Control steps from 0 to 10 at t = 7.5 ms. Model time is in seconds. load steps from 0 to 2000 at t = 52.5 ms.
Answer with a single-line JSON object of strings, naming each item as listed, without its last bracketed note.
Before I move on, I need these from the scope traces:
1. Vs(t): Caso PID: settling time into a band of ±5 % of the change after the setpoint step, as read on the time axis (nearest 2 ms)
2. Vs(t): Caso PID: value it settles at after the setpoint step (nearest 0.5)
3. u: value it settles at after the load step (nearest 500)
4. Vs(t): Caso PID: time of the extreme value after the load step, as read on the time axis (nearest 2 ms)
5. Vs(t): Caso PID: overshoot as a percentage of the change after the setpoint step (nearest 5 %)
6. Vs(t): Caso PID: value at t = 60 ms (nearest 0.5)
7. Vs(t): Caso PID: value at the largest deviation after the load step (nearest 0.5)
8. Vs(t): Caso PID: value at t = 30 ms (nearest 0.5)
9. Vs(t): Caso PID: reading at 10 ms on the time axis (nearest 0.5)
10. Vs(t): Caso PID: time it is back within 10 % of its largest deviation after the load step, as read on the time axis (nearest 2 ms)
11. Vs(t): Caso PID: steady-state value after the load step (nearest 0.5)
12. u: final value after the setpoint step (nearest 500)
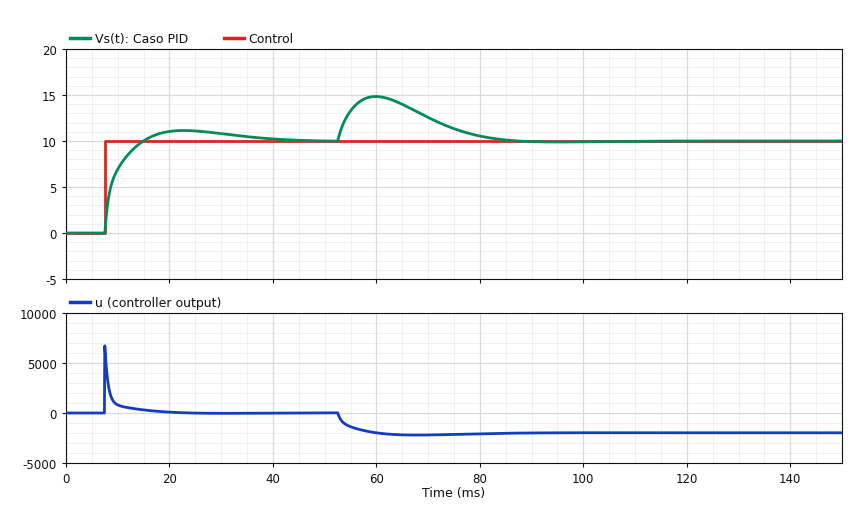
{"Vs(t): Caso PID: settling time into a band of ±5 % of the change after the setpoint step, as read on the time axis": "34 ms", "Vs(t): Caso PID: value it settles at after the setpoint step": "10.0", "u: value it settles at after the load step": "-2000", "Vs(t): Caso PID: time of the extreme value after the load step, as read on the time axis": "60 ms", "Vs(t): Caso PID: overshoot as a percentage of the change after the setpoint step": "10 %", "Vs(t): Caso PID: value at t = 60 ms": "15.0", "Vs(t): Caso PID: value at the largest deviation after the load step": "15.0", "Vs(t): Caso PID: value at t = 30 ms": "11.0", "Vs(t): Caso PID: reading at 10 ms on the time axis": "7.0", "Vs(t): Caso PID: time it is back within 10 % of its largest deviation after the load step, as read on the time axis": "80 ms", "Vs(t): Caso PID: steady-state value after the load step": "10.0", "u: final value after the setpoint step": "0"}
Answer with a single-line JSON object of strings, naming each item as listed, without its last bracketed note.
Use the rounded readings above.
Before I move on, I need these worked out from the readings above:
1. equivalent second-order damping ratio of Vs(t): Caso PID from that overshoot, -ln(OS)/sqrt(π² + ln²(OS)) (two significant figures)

{"equivalent second-order damping ratio of Vs(t): Caso PID from that overshoot, -ln(OS)/sqrt(π² + ln²(OS))": "0.59"}
